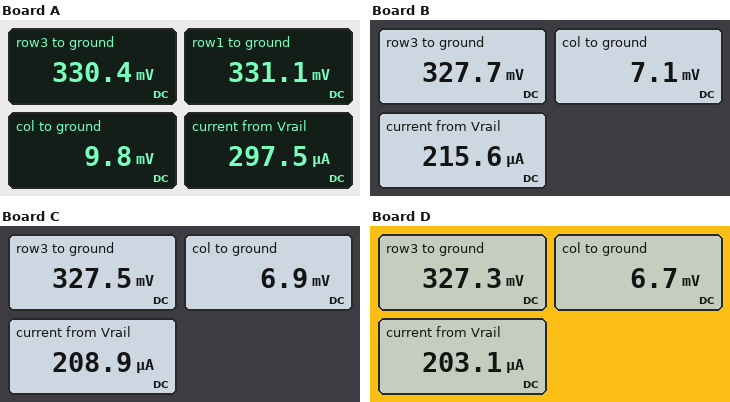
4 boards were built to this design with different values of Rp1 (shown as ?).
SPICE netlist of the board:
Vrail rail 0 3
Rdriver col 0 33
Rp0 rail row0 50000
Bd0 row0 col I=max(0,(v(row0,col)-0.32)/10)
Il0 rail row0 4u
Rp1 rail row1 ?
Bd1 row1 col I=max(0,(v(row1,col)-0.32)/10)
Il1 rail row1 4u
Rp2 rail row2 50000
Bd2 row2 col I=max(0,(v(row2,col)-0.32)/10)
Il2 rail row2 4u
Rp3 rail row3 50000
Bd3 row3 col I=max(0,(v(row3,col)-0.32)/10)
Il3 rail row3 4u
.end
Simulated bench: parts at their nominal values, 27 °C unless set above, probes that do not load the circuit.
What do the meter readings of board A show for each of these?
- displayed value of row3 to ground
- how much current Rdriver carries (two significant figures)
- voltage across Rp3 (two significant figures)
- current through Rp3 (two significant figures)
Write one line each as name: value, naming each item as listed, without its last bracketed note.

displayed value of row3 to ground: 330.4 mV
how much current Rdriver carries: 300 µA
voltage across Rp3: 2.7 V
current through Rp3: 53 µA
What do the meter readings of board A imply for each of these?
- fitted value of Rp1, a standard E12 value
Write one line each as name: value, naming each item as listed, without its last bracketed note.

fitted value of Rp1, a standard E12 value: 22 kΩ
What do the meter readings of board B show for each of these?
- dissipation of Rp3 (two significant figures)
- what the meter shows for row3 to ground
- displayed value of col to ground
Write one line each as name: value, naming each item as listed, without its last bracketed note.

dissipation of Rp3: 140 µW
what the meter shows for row3 to ground: 327.7 mV
displayed value of col to ground: 7.1 mV
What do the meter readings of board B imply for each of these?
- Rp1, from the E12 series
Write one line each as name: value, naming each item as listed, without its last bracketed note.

Rp1, from the E12 series: 68 kΩ
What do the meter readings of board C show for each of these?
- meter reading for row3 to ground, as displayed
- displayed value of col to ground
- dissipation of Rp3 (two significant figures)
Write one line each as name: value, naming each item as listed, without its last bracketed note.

meter reading for row3 to ground, as displayed: 327.5 mV
displayed value of col to ground: 6.9 mV
dissipation of Rp3: 140 µW
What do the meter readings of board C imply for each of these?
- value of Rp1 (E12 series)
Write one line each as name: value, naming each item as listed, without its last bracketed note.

value of Rp1: 82 kΩ
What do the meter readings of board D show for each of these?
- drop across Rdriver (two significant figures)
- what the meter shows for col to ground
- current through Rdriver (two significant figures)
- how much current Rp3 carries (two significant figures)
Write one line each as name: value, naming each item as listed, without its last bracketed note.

drop across Rdriver: 6.7 mV
what the meter shows for col to ground: 6.7 mV
current through Rdriver: 200 µA
how much current Rp3 carries: 53 µA
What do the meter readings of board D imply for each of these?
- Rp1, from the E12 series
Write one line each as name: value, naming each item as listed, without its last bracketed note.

Rp1, from the E12 series: 100 kΩ
